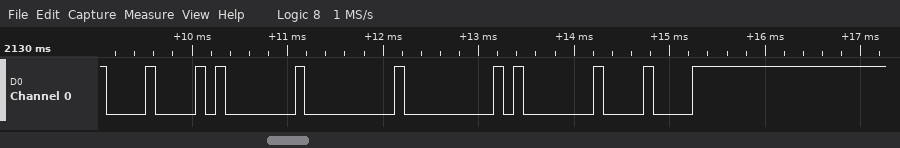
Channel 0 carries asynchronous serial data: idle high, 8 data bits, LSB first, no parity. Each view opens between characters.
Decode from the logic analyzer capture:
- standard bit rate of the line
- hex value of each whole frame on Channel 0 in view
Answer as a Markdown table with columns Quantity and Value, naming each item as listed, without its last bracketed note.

| Quantity | Value |
|---|---|
| standard bit rate of the line | 9600 baud |
| hex value of each whole frame on Channel 0 in view | 08, 01, 00, 00, 01, 08 |
